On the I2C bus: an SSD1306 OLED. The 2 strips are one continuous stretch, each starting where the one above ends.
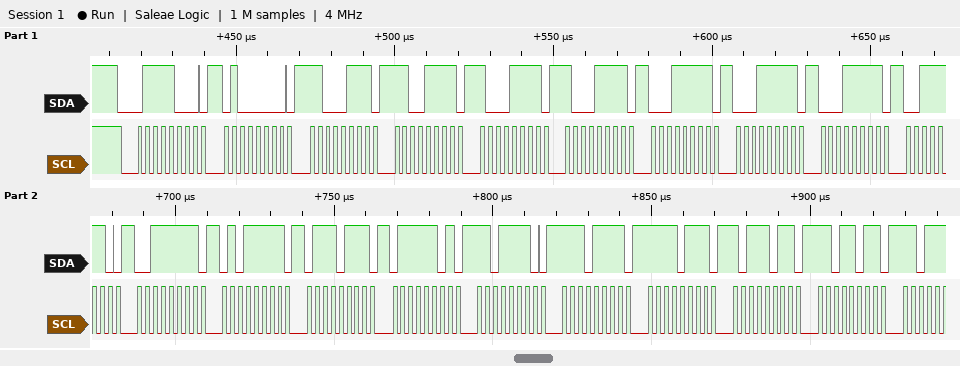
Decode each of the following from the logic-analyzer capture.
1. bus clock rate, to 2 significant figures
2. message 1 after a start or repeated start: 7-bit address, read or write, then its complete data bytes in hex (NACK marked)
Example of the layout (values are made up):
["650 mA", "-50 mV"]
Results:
["400 kHz", "0x3C write: 40 C7 CF 8F 8F 1F 1F 1F 3E 3F 5F 77 7D DE EF F7 BB DB"]
